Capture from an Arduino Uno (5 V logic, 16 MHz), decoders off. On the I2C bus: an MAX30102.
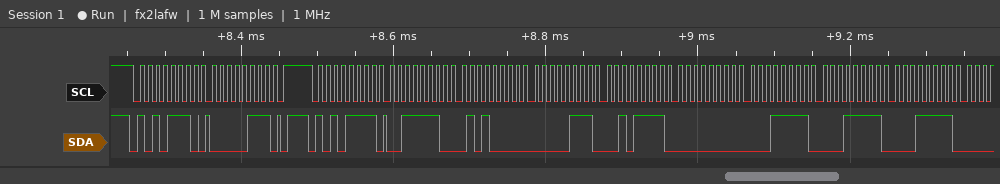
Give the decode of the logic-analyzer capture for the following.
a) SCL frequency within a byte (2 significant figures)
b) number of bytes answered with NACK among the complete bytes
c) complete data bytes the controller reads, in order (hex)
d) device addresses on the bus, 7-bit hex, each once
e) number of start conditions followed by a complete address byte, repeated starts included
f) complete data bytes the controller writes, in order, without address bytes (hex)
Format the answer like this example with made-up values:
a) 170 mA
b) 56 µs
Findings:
a) 100 kHz
b) 0
c) 3E 50 07 2F 00 1F 1F 1F
d) 0x57
e) 2
f) 07
